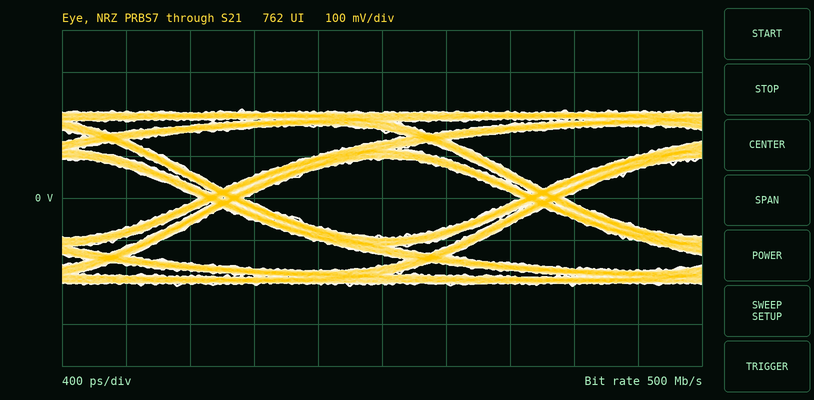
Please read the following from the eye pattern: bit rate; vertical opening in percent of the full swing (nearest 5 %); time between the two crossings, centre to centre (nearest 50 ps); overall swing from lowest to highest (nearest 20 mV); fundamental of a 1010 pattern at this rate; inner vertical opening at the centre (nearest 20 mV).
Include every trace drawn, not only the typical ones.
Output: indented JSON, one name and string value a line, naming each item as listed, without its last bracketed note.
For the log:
{
  "bit rate": "500 Mb/s",
  "vertical opening in percent of the full swing": "45 %",
  "time between the two crossings, centre to centre": "2.00 ns",
  "overall swing from lowest to highest": "420 mV",
  "fundamental of a 1010 pattern at this rate": "250 MHz",
  "inner vertical opening at the centre": "180 mV"
}
